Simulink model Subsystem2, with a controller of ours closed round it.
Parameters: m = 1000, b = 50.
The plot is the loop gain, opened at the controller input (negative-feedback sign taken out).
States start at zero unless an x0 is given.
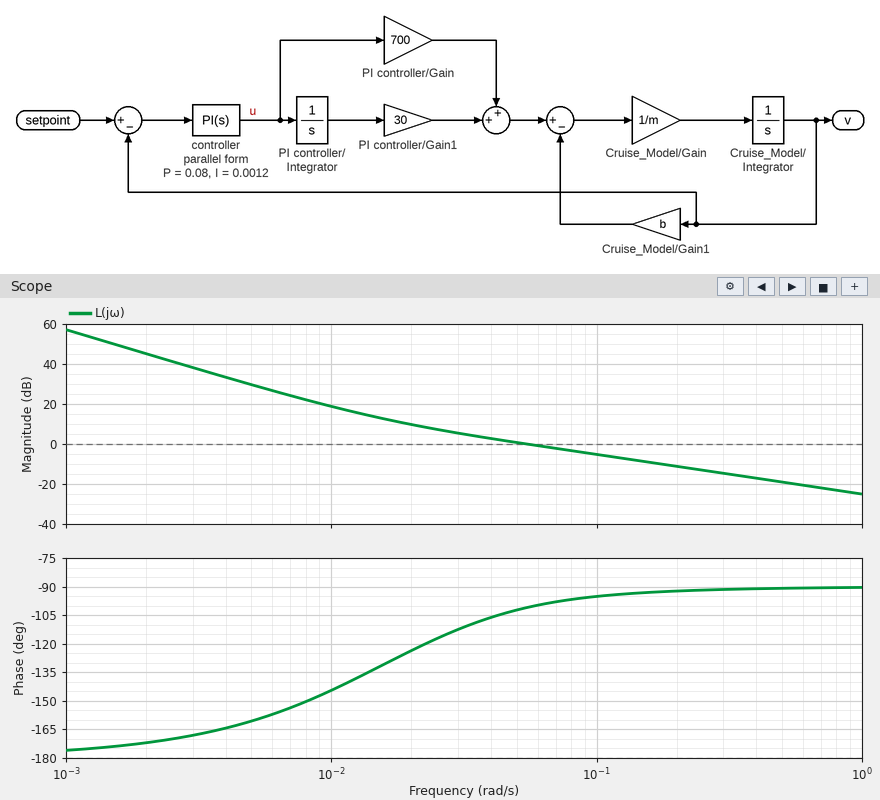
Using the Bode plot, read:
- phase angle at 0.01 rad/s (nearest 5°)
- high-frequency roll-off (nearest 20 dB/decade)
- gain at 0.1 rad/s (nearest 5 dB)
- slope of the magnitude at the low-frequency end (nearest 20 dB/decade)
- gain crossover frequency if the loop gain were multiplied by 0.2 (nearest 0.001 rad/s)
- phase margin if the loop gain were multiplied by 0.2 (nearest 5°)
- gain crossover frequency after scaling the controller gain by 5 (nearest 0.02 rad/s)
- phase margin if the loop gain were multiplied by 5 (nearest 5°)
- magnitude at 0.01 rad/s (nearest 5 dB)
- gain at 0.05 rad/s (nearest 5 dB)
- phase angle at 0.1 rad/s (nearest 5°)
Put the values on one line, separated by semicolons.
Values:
-145°; -20 dB/decade; -5 dB; -40 dB/decade; 0.014 rad/s; 45°; 0.28 rad/s; 90°; 20 dB; 0 dB; -95°
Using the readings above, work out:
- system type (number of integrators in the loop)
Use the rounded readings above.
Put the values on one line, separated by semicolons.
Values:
2
